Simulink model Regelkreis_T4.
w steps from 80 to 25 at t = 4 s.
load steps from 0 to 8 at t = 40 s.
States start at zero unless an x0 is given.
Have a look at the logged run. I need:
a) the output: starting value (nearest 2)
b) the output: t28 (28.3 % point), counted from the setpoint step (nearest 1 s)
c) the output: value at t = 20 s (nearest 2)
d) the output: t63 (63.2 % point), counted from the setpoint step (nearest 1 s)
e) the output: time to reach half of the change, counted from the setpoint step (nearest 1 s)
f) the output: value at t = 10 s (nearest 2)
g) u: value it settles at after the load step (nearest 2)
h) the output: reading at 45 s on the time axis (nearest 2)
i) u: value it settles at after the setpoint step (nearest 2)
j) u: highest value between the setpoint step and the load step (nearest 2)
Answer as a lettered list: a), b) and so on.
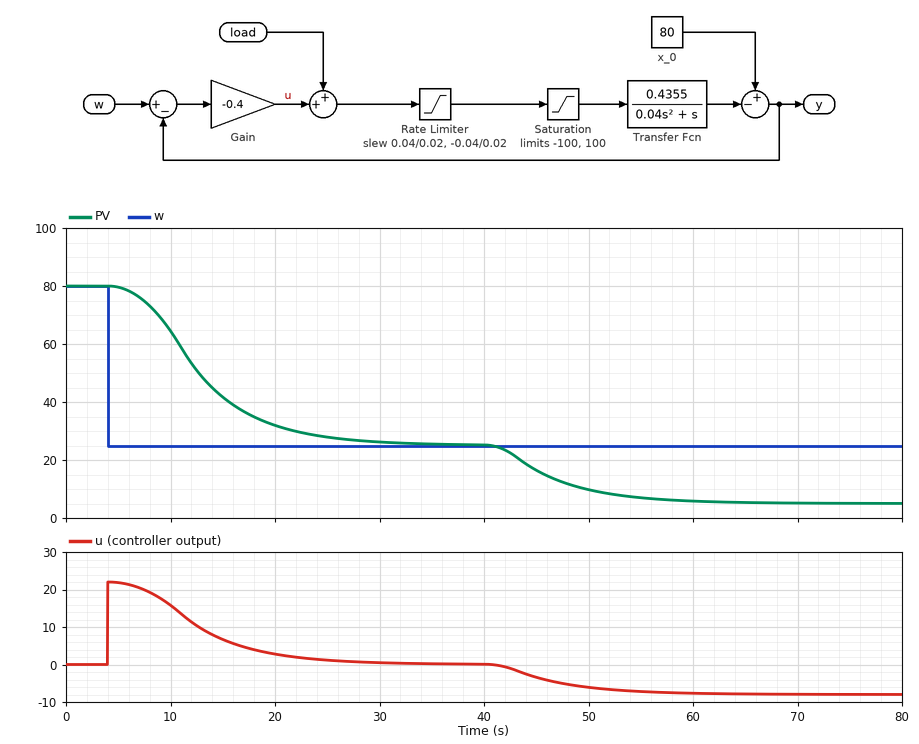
a) 80
b) 6 s
c) 32
d) 10 s
e) 8 s
f) 64
g) -8
h) 16
i) 0
j) 22
